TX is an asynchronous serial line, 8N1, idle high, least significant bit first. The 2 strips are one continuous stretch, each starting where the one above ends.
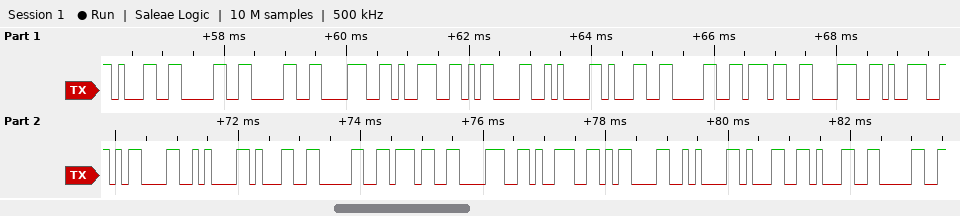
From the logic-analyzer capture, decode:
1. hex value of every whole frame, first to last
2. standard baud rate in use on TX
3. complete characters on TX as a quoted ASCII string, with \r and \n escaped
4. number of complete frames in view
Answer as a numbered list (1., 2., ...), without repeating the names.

1. 31 30 30 38 39 0D 0A 31 30 37 38 39 0D 0A 31 30 37 38 39 0D 0A 31 31 30
2. 9600 baud
3. "10089\r\n10789\r\n10789\r\n110"
4. 24
